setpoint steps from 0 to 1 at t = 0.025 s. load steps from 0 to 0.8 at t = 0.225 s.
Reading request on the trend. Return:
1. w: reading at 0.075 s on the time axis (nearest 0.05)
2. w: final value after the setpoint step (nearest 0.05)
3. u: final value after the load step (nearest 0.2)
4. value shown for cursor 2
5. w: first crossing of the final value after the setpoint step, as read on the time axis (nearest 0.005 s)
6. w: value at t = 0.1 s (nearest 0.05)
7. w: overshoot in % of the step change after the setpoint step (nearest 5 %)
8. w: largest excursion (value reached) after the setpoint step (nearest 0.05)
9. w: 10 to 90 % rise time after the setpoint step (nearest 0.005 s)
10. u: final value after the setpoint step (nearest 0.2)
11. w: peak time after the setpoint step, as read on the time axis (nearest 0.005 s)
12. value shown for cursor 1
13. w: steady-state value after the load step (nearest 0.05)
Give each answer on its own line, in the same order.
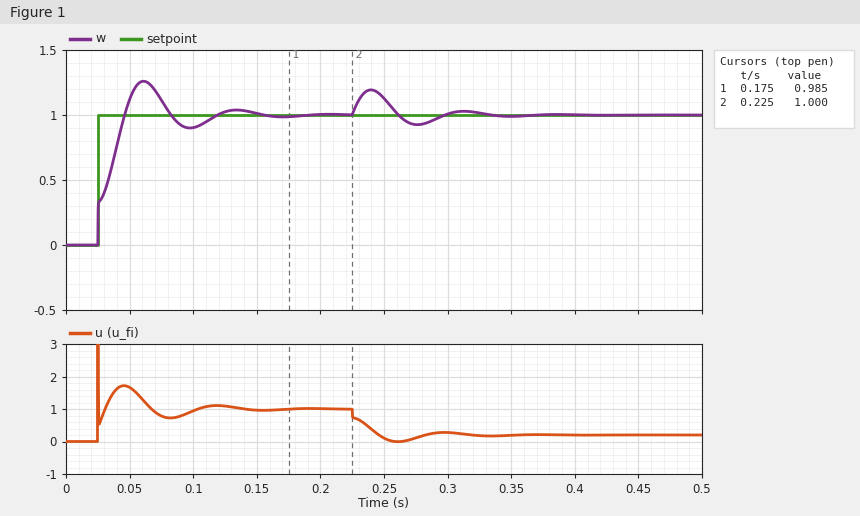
1.10
1.00
0.2
1.000
0.045 s
0.90
25 %
1.25
0.020 s
1.0
0.060 s
0.985
1.00
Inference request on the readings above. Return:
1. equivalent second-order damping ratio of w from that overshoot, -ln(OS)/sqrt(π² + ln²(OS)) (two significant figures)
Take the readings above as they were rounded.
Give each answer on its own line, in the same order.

0.40
